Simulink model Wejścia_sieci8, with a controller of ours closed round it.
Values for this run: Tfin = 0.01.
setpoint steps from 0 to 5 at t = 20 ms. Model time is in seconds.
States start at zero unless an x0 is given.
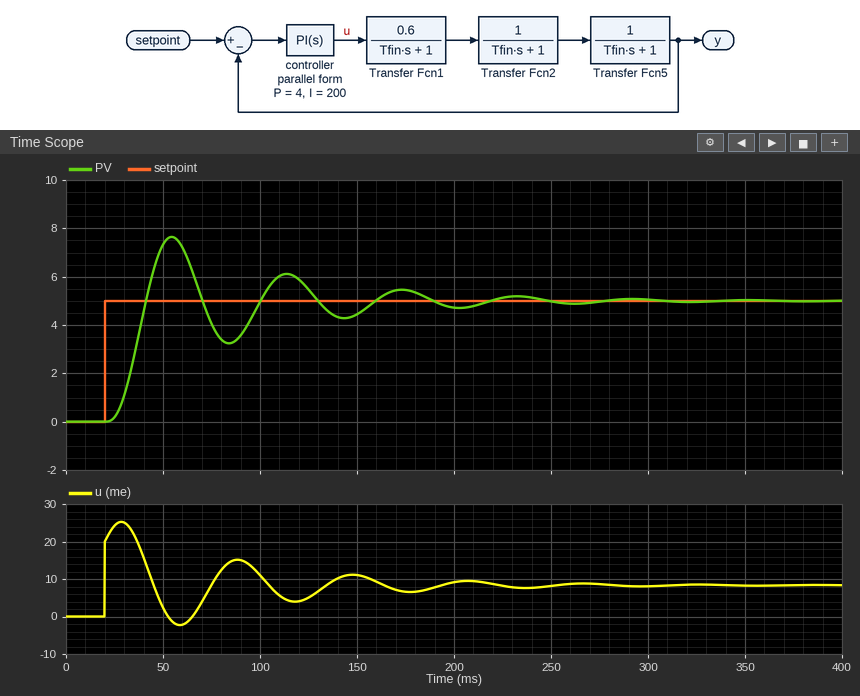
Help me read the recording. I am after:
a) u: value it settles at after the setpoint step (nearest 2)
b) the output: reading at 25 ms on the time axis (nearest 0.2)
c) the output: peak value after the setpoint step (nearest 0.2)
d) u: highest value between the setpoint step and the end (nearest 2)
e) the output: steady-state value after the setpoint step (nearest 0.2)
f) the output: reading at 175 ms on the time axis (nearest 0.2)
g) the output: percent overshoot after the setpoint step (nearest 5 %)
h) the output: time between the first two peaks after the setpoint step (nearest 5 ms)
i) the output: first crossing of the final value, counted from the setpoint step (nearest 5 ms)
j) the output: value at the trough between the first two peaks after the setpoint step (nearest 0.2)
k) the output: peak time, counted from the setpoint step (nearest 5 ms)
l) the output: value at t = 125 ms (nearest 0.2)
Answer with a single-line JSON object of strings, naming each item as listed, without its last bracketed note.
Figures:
{"u: value it settles at after the setpoint step": "8", "the output: reading at 25 ms on the time axis": "0.2", "the output: peak value after the setpoint step": "7.6", "u: highest value between the setpoint step and the end": "26", "the output: steady-state value after the setpoint step": "5.0", "the output: reading at 175 ms on the time axis": "5.4", "the output: percent overshoot after the setpoint step": "55 %", "the output: time between the first two peaks after the setpoint step": "60 ms", "the output: first crossing of the final value, counted from the setpoint step": "20 ms", "the output: value at the trough between the first two peaks after the setpoint step": "3.2", "the output: peak time, counted from the setpoint step": "35 ms", "the output: value at t = 125 ms": "5.4"}
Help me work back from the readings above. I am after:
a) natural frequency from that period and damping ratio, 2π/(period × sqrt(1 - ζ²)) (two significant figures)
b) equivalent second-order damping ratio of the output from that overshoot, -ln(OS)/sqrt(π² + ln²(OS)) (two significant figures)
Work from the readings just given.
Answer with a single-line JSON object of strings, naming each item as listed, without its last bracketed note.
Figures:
{"natural frequency from that period and damping ratio, 2π/(period × sqrt(1 - ζ²))": "0.11 rad/ms", "equivalent second-order damping ratio of the output from that overshoot, -ln(OS)/sqrt(π² + ln²(OS))": "0.19"}
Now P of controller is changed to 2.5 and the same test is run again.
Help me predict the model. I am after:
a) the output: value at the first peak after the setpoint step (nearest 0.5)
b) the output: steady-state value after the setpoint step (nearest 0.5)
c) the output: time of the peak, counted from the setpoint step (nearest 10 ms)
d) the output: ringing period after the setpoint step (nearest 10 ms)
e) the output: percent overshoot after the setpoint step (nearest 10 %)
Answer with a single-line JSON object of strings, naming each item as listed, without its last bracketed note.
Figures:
{"the output: value at the first peak after the setpoint step": "8.0", "the output: steady-state value after the setpoint step": "5.0", "the output: time of the peak, counted from the setpoint step": "40 ms", "the output: ringing period after the setpoint step": "70 ms", "the output: percent overshoot after the setpoint step": "60 %"}
